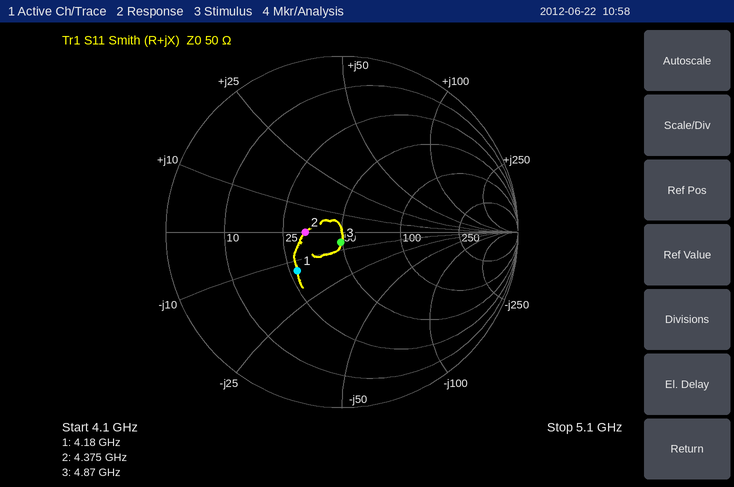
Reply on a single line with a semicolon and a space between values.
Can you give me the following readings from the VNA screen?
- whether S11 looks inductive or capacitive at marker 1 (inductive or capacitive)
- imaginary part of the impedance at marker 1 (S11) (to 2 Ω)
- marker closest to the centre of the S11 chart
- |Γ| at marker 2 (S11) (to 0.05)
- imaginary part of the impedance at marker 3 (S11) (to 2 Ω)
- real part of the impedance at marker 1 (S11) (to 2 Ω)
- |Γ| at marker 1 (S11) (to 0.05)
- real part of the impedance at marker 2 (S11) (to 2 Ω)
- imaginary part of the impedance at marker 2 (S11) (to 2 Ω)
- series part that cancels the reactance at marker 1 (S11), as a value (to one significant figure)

capacitive; -14 Ω; marker 3; 0.20; -6 Ω; 28 Ω; 0.35; 32 Ω; 0 Ω; 500 pH
